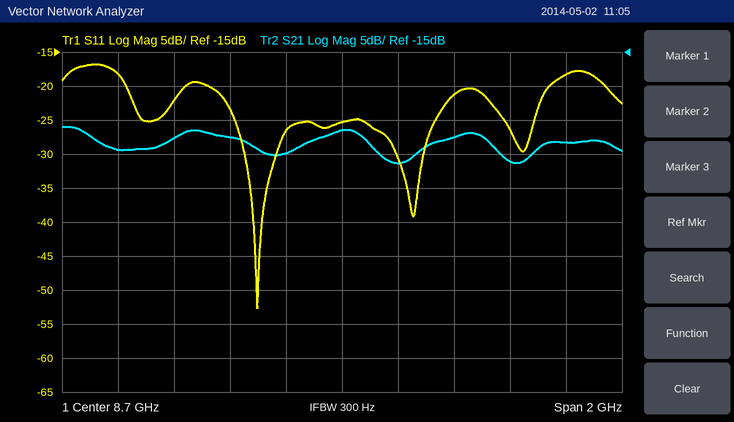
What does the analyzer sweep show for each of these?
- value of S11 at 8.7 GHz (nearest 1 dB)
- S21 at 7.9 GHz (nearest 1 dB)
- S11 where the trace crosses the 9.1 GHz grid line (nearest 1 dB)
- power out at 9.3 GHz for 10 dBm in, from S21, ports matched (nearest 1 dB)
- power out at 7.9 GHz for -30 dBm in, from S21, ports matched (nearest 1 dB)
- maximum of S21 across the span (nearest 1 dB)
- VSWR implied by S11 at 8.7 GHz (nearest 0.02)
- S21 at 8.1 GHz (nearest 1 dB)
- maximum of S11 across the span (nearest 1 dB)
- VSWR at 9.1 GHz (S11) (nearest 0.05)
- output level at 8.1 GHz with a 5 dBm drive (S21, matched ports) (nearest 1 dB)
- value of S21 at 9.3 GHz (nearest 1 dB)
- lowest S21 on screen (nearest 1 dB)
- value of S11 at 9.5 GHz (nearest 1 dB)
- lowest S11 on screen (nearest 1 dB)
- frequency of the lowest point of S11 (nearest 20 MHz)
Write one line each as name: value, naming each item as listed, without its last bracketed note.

value of S11 at 8.7 GHz: -25 dB
S21 at 7.9 GHz: -29 dB
S11 where the trace crosses the 9.1 GHz grid line: -21 dB
power out at 9.3 GHz for 10 dBm in, from S21, ports matched: -21 dBm
power out at 7.9 GHz for -30 dBm in, from S21, ports matched: -59 dBm
maximum of S21 across the span: -26 dB
VSWR implied by S11 at 8.7 GHz: 1.12
S21 at 8.1 GHz: -28 dB
maximum of S11 across the span: -17 dB
VSWR at 9.1 GHz (S11): 1.20
output level at 8.1 GHz with a 5 dBm drive (S21, matched ports): -23 dBm
value of S21 at 9.3 GHz: -31 dB
lowest S21 on screen: -31 dB
value of S11 at 9.5 GHz: -18 dB
lowest S11 on screen: -53 dB
frequency of the lowest point of S11: 8.40 GHz
